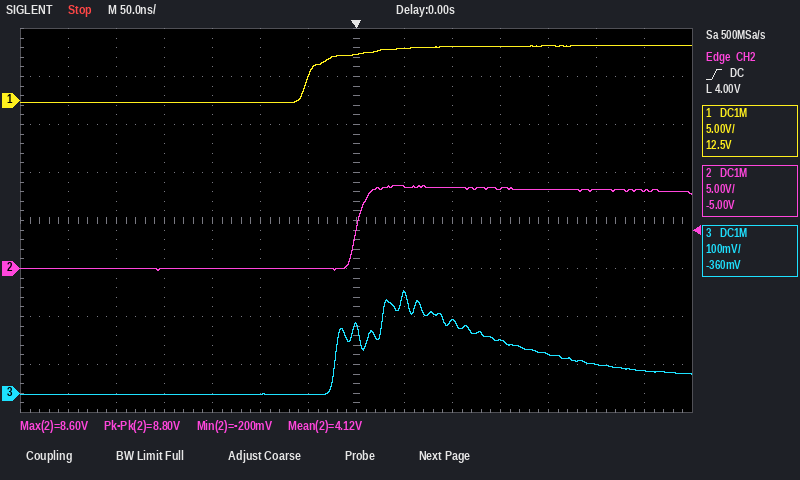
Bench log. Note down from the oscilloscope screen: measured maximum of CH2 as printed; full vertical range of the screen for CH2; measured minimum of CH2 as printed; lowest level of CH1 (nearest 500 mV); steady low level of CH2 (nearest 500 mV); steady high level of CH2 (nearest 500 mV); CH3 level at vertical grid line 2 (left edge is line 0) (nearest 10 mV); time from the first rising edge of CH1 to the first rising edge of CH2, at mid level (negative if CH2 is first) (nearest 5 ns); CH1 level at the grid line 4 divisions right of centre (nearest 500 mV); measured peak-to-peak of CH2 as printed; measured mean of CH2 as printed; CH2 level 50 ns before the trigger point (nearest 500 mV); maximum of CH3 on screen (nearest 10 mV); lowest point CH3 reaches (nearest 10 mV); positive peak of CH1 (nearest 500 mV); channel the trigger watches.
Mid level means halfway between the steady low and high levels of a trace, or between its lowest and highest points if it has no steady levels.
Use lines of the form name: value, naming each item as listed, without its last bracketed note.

measured maximum of CH2 as printed: 8.60 V
full vertical range of the screen for CH2: 40 V
measured minimum of CH2 as printed: -200 mV
lowest level of CH1: 0.0 V
steady low level of CH2: 0.0 V
steady high level of CH2: 8.0 V
CH3 level at vertical grid line 2 (left edge is line 0): 0 mV
time from the first rising edge of CH1 to the first rising edge of CH2, at mid level (negative if CH2 is first): +50 ns
CH1 level at the grid line 4 divisions right of centre: 5.5 V
measured peak-to-peak of CH2 as printed: 8.80 V
measured mean of CH2 as printed: 4.12 V
CH2 level 50 ns before the trigger point: 0.0 V
maximum of CH3 on screen: 210 mV
lowest point CH3 reaches: 0 mV
positive peak of CH1: 5.5 V
channel the trigger watches: CH2
